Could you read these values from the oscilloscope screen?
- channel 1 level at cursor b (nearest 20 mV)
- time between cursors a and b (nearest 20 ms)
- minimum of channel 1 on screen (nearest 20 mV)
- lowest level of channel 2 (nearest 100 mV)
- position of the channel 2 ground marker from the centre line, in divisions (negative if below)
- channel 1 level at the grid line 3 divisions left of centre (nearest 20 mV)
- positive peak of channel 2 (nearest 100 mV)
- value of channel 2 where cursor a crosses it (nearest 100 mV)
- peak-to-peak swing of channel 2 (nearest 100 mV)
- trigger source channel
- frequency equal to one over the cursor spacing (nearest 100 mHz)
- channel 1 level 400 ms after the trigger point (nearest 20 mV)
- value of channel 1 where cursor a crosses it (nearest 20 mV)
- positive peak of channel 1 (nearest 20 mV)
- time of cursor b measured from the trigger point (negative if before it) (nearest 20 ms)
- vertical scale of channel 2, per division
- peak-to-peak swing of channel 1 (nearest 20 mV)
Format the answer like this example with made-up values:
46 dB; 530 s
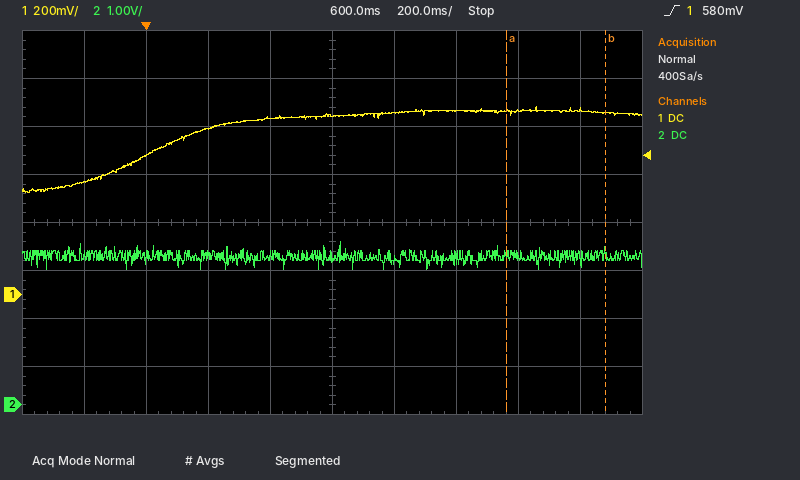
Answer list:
760 mV; 320 ms; 420 mV; 2.8 V; -3.8 div; 580 mV; 3.4 V; 3.1 V; 600 mV; channel 1; 3.1 Hz; 740 mV; 760 mV; 780 mV; +1.48 s; 1 V; 360 mV
